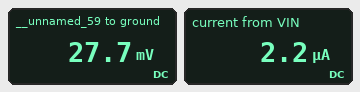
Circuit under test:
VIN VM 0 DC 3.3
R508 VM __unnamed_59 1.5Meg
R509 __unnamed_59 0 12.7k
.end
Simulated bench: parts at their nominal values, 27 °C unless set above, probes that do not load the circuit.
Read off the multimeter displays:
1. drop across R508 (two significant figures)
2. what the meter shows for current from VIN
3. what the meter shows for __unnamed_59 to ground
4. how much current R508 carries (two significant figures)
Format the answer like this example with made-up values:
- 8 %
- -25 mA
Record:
- 3.3 V
- 2.2 µA
- 27.7 mV
- 2.2 µA
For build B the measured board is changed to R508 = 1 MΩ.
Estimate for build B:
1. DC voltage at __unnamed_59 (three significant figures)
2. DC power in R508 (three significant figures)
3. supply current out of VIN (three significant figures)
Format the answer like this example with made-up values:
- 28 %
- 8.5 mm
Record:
- 41.4 mV
- 10.6 µW
- 3.26 µA
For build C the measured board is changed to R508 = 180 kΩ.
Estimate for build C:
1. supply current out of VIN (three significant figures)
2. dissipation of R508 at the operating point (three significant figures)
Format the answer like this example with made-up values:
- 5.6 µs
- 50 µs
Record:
- 17.1 µA
- 52.8 µW
